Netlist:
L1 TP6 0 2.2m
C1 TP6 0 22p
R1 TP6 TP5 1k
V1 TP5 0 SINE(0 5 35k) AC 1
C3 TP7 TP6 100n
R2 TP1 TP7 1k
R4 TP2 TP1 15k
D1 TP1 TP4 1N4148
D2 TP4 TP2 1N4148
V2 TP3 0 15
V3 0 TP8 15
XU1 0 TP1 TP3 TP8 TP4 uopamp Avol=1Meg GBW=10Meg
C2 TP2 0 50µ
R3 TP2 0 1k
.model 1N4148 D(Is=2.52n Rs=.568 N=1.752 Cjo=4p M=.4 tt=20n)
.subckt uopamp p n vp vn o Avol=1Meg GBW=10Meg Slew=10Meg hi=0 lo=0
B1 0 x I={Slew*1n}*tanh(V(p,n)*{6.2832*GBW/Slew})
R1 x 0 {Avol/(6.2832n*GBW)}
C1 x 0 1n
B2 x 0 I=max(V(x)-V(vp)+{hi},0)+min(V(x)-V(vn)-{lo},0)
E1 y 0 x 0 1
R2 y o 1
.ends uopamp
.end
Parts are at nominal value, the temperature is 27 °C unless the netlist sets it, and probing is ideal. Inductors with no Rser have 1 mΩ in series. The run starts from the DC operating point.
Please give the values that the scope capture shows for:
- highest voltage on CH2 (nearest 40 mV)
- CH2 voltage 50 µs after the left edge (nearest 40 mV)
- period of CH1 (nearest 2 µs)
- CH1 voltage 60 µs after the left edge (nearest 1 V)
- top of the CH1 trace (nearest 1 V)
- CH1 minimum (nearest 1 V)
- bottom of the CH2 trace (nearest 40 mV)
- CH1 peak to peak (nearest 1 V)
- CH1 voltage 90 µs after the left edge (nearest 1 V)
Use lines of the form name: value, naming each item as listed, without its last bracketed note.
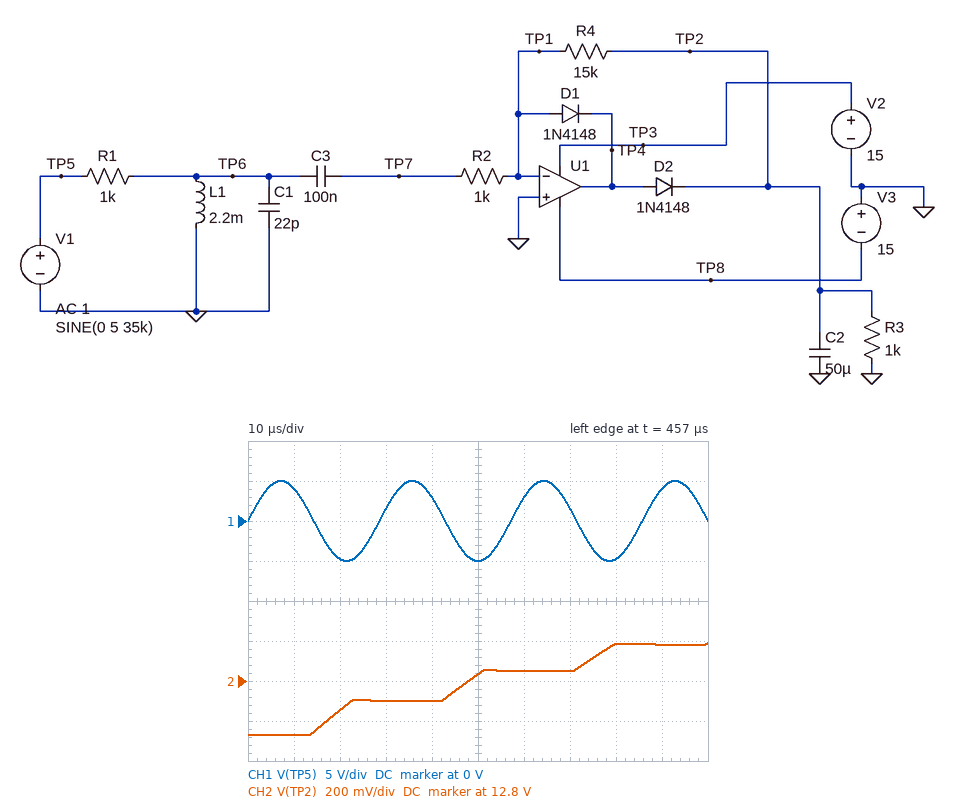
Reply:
highest voltage on CH2: 13.00 V
CH2 voltage 50 µs after the left edge: 12.84 V
period of CH1: 28 µs
CH1 voltage 60 µs after the left edge: 3 V
top of the CH1 trace: 5 V
CH1 minimum: -5 V
bottom of the CH2 trace: 12.52 V
CH1 peak to peak: 10 V
CH1 voltage 90 µs after the left edge: 4 V
